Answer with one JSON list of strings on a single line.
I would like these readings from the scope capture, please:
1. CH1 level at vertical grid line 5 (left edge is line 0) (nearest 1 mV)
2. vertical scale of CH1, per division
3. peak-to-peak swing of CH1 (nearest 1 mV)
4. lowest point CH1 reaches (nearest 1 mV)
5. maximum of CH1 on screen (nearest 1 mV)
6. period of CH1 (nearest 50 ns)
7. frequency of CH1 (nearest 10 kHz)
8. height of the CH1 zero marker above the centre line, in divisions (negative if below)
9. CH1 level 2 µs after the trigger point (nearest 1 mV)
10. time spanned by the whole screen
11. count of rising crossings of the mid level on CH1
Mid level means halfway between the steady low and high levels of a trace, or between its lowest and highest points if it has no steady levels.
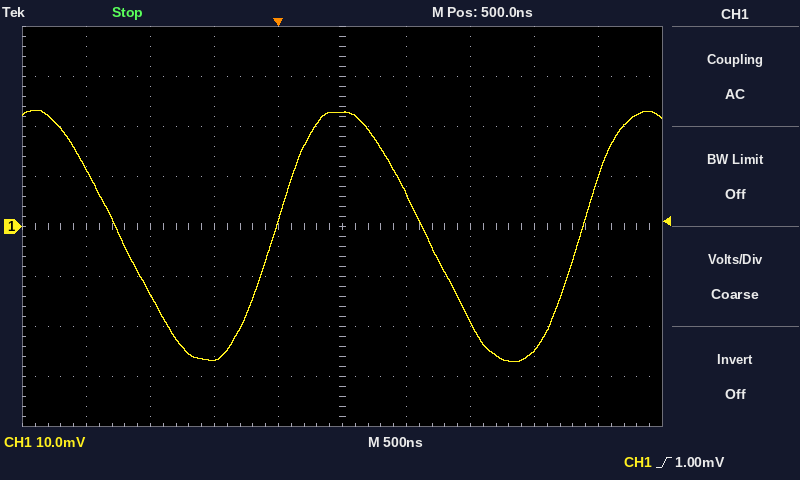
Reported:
["23 mV", "10 mV", "50 mV", "-27 mV", "23 mV", "2.40 µs", "420 kHz", "0.0 div", "-25 mV", "5 µs", "2"]
